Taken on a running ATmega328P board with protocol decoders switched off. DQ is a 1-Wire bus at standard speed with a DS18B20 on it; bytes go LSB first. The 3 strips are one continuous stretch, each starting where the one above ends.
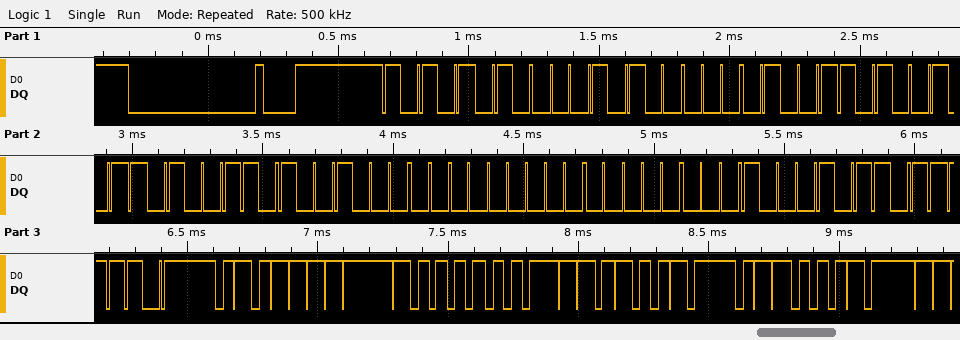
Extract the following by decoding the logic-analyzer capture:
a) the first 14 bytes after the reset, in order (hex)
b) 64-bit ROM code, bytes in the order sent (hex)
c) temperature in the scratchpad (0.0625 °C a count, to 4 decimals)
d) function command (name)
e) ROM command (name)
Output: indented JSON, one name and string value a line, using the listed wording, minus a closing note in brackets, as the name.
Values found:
{
  "the first 14 bytes after the reset, in order": "55 28 90 A5 65 09 00 00 D1 BE FA 01 4B 46",
  "64-bit ROM code, bytes in the order sent": "28 90 A5 65 09 00 00 D1",
  "temperature in the scratchpad": "31.6250 °C",
  "function command": "Read Scratchpad",
  "ROM command": "Match ROM"
}
